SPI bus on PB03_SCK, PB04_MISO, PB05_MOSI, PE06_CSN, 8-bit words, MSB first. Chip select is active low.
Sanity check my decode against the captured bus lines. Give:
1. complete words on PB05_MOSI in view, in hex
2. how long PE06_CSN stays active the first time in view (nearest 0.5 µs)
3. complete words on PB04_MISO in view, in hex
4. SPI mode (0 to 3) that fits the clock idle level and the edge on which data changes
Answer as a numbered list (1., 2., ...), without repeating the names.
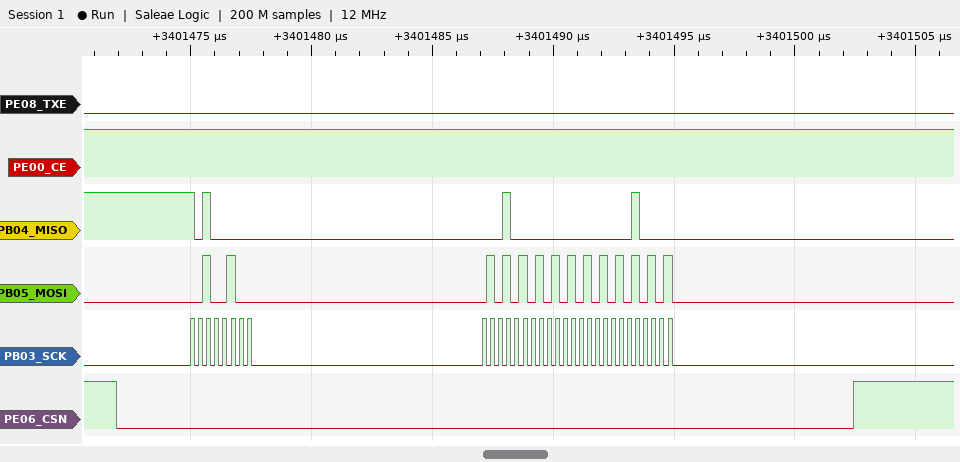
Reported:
1. 24, 55, 55, 55
2. 30.5 µs
3. A0, 10, 00, 10
4. 0
